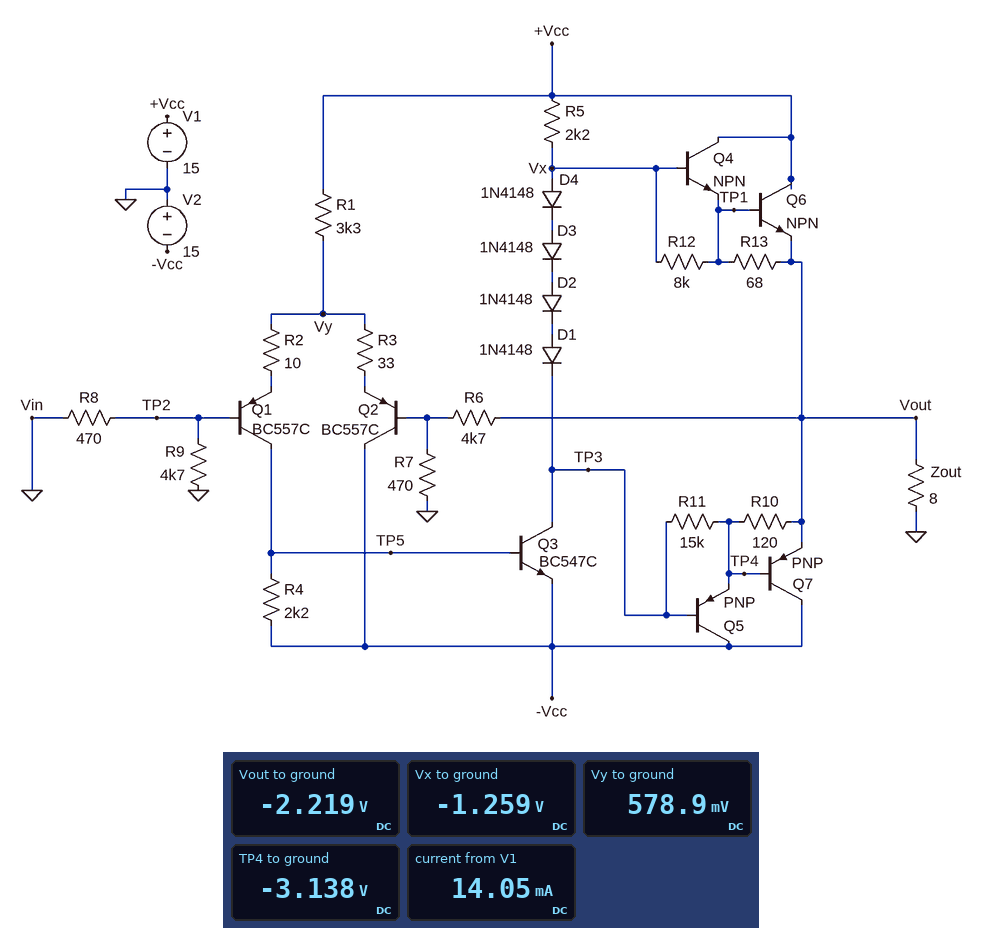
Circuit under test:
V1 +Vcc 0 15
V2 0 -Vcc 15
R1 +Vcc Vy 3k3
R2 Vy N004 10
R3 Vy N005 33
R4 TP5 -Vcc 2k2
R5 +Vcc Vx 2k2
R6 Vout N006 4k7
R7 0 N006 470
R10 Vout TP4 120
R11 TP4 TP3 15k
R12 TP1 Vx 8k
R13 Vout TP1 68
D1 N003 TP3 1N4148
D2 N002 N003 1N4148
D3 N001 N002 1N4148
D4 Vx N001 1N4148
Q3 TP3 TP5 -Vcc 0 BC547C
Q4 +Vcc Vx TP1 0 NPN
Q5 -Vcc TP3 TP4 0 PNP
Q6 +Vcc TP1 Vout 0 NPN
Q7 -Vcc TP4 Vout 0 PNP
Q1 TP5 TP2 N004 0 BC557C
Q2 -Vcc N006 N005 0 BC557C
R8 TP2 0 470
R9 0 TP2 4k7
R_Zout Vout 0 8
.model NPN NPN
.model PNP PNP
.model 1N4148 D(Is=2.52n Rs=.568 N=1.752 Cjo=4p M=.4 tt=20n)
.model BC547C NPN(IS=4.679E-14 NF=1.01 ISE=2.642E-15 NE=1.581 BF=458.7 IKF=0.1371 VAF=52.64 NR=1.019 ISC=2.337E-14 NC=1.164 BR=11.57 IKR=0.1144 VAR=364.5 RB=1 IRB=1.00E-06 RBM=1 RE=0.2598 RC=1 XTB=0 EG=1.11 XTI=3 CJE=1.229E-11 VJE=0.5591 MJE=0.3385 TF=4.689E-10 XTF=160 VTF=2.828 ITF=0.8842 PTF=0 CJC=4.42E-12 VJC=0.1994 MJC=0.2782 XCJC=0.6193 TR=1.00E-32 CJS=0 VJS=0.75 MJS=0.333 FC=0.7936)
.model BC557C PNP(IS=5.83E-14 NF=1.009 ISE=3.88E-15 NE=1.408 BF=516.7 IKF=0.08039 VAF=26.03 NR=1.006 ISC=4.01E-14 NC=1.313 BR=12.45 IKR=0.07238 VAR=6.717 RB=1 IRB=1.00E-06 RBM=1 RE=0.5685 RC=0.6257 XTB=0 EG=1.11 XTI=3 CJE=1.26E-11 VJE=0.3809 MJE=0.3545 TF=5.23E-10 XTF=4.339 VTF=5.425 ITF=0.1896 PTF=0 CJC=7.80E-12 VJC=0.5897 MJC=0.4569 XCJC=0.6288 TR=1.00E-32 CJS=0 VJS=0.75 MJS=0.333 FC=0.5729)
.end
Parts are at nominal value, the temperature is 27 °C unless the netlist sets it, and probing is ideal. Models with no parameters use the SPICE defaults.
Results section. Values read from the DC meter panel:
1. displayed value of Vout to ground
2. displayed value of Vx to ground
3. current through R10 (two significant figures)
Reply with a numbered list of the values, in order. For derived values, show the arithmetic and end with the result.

1. -2.219 V
2. -1.259 V
3. (-2.219 V - (-3.138 V)) / 120 Ω = 7.7 mA
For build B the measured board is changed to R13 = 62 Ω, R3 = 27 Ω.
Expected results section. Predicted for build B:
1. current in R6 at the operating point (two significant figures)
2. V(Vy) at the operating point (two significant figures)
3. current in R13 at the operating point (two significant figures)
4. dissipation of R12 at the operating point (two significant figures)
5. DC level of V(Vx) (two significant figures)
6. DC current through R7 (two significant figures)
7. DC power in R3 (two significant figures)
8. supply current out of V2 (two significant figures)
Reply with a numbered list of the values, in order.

1. 380 µA
2. 580 mV
3. 2.6 mA
4. 80 µW
5. -990 mV
6. 370 µA
7. 440 µW
8. 260 mA
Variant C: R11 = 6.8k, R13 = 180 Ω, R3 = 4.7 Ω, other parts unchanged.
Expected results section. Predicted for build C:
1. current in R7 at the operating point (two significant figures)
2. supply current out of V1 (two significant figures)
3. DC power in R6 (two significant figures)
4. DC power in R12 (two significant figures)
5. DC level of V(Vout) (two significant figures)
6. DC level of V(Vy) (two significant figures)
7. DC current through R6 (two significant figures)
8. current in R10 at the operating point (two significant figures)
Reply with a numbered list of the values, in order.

1. 180 µA
2. 12 mA
3. 160 µW
4. 75 µW
5. -960 mV
6. 580 mV
7. 190 µA
8. 7.5 mA
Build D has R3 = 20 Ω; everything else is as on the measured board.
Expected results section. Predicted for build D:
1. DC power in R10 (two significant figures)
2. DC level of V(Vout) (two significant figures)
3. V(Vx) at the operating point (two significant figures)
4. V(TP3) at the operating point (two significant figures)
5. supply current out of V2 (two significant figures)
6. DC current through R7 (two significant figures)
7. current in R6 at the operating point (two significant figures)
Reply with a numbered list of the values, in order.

1. 6.9 mW
2. -1.6 V
3. -680 mV
4. -3.4 V
5. 220 mA
6. 310 µA
7. 320 µA
